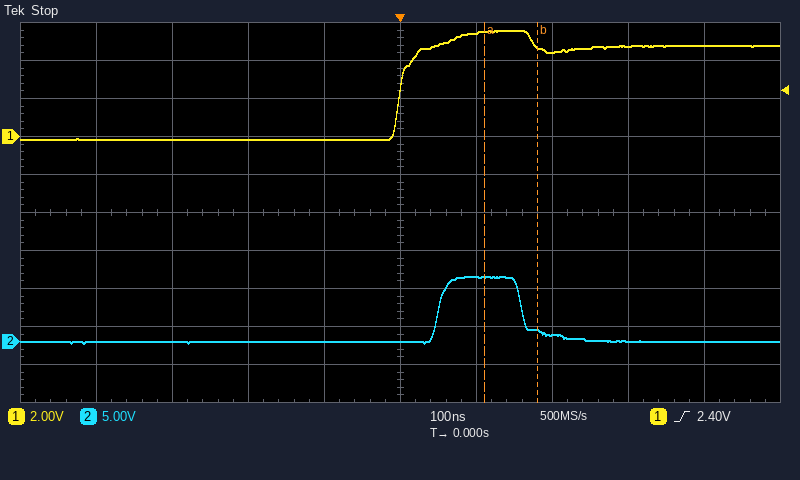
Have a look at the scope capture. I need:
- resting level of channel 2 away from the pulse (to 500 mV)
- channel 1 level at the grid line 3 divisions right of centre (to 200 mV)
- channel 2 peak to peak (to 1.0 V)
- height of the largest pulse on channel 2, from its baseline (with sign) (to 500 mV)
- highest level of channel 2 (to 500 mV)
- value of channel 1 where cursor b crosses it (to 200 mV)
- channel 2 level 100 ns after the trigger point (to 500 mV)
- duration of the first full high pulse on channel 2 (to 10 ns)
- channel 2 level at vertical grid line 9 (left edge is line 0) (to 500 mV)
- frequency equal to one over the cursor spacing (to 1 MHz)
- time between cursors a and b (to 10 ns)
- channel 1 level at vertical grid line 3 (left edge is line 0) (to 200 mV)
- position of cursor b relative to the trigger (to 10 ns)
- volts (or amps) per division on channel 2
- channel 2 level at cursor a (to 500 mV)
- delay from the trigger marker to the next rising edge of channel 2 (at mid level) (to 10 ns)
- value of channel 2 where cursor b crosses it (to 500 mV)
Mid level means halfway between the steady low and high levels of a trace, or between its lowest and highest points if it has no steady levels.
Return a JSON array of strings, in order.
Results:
["0.0 V", "4.8 V", "9.0 V", "+8.5 V", "8.5 V", "4.8 V", "8.5 V", "110 ns", "0.0 V", "14 MHz", "70 ns", "-200 mV", "+180 ns", "5 V", "8.5 V", "50 ns", "1.5 V"]
